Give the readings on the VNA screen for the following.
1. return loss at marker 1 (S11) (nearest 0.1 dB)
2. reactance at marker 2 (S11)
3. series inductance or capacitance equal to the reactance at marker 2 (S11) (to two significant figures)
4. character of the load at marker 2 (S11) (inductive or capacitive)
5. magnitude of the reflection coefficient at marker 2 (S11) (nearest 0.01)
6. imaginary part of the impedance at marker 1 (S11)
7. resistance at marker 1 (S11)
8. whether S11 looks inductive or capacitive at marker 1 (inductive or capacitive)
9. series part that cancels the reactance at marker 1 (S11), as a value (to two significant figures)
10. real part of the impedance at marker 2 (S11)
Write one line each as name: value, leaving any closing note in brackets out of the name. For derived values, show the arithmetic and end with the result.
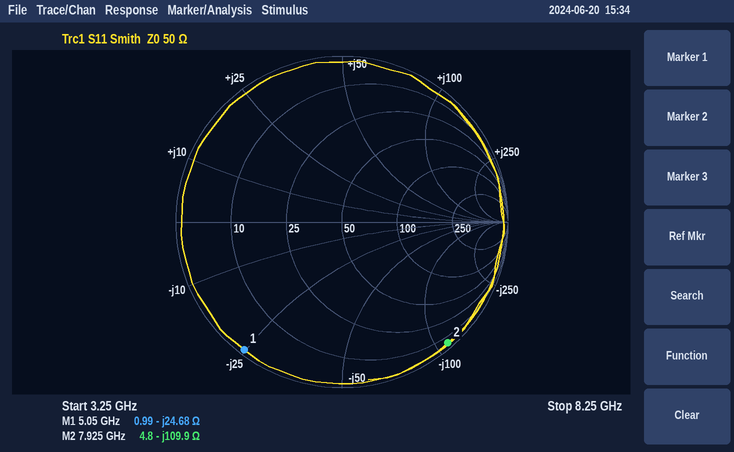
return loss at marker 1 (S11): 0.3 dB
reactance at marker 2: -109.9 Ω
series inductance or capacitance equal to the reactance at marker 2 (S11): C = 1/(2π × 7.925 GHz × 109.9 Ω) ≈ 183 fF, so 180 fF to two significant figures
character of the load at marker 2 (S11): capacitive
magnitude of the reflection coefficient at marker 2 (S11): 0.97
imaginary part of the impedance at marker 1: -24.68 Ω
resistance at marker 1: 0.99 Ω
whether S11 looks inductive or capacitive at marker 1: capacitive
series part that cancels the reactance at marker 1 (S11), as a value: L = 24.68 Ω/(2π × 5.05 GHz) ≈ 778 pH, so 780 pH to two significant figures
real part of the impedance at marker 2: 4.8 Ω
